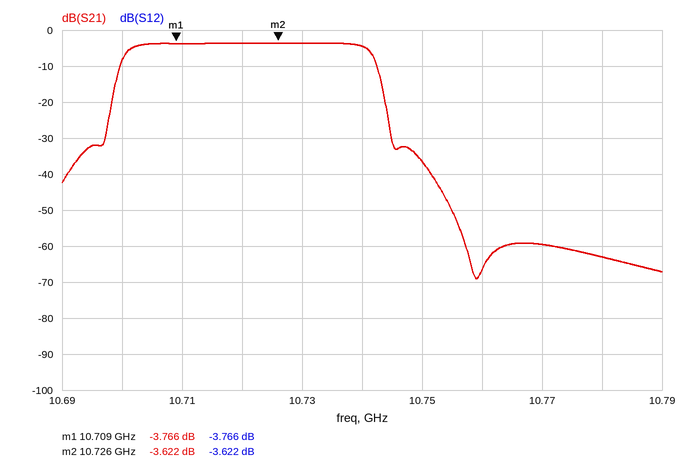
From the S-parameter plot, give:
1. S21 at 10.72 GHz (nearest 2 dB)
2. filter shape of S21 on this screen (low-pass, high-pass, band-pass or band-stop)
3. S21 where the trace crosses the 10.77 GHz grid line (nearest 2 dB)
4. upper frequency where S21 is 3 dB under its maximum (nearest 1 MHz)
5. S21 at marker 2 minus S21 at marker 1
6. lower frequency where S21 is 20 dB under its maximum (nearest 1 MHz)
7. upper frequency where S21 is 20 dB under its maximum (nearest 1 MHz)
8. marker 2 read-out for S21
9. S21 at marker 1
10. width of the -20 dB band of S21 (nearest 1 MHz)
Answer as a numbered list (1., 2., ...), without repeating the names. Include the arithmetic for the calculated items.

1. -4 dB
2. band-pass
3. -60 dB
4. 10.742 GHz
5. -3.622 − (-3.766) = 0.144 dB
6. 10.698 GHz
7. 10.744 GHz
8. -3.622 dB
9. -3.766 dB
10. 10.744 GHz − 10.698 GHz = 46 MHz
